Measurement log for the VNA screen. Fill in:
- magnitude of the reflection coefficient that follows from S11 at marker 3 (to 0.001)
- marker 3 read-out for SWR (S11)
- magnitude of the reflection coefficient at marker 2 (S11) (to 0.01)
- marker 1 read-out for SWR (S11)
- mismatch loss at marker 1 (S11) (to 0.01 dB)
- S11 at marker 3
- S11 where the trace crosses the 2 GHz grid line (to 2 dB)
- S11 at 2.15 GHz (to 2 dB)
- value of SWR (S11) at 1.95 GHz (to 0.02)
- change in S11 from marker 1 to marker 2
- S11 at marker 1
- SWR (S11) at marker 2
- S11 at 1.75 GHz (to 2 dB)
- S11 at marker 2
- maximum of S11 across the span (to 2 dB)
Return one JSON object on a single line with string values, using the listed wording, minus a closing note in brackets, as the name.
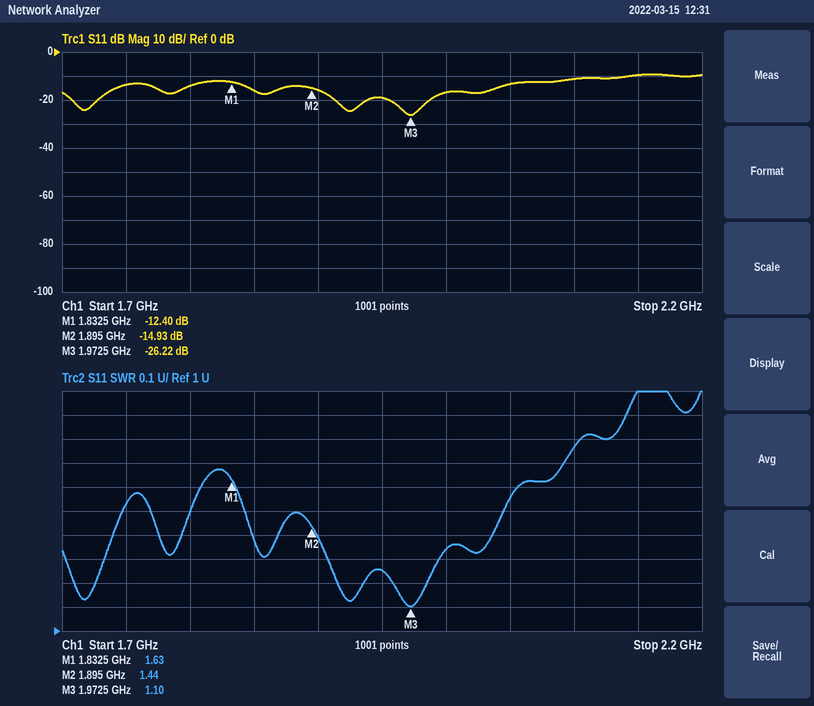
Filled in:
{"magnitude of the reflection coefficient that follows from S11 at marker 3": "0.049", "marker 3 read-out for SWR": "1.10", "magnitude of the reflection coefficient at marker 2 (S11)": "0.18", "marker 1 read-out for SWR": "1.63", "mismatch loss at marker 1 (S11)": "0.26 dB", "S11 at marker 3": "-26.22 dB", "S11 where the trace crosses the 2 GHz grid line": "-16 dB", "S11 at 2.15 GHz": "-10 dB", "value of SWR (S11) at 1.95 GHz": "1.26", "change in S11 from marker 1 to marker 2": "-2.53 dB", "S11 at marker 1": "-12.40 dB", "SWR (S11) at marker 2": "1.44", "S11 at 1.75 GHz": "-14 dB", "S11 at marker 2": "-14.93 dB", "maximum of S11 across the span": "-10 dB"}
